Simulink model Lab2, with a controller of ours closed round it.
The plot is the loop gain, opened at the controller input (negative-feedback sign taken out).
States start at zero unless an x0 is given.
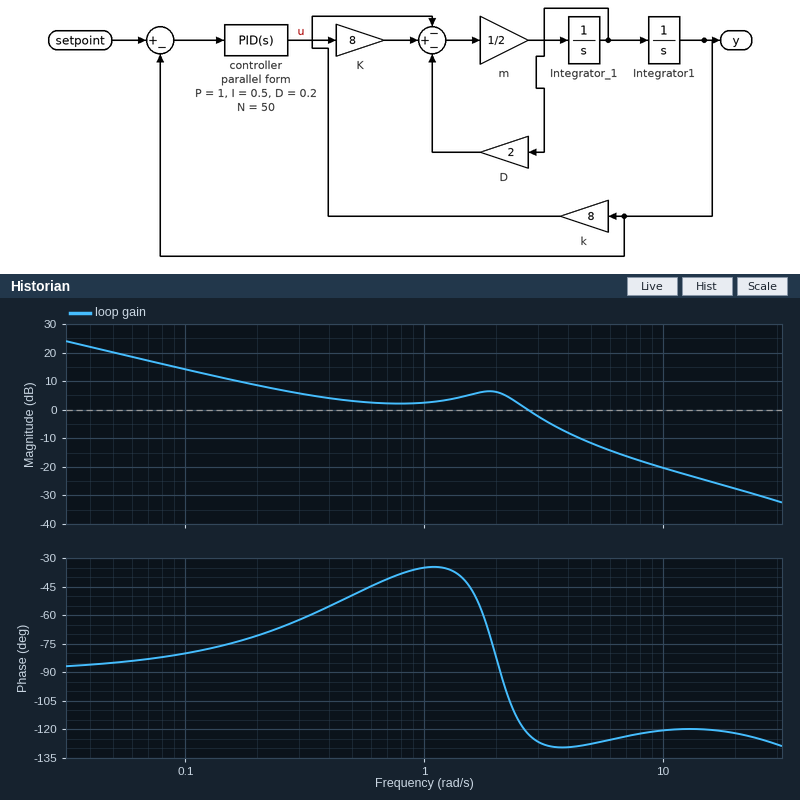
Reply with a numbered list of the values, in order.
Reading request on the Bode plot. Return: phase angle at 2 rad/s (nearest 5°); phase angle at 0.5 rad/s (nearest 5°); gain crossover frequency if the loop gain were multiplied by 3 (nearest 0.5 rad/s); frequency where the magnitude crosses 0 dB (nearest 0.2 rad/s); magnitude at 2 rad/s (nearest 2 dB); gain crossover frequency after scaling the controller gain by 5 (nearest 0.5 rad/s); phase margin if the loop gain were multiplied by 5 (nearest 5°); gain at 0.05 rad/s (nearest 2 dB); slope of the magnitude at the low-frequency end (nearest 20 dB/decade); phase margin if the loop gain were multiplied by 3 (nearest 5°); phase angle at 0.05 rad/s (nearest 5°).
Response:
1. -80°
2. -50°
3. 4.5 rad/s
4. 2.8 rad/s
5. 6 dB
6. 6.0 rad/s
7. 55°
8. 20 dB
9. -20 dB/decade
10. 50°
11. -85°
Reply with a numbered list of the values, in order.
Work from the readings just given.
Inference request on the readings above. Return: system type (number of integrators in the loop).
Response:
1. 1
